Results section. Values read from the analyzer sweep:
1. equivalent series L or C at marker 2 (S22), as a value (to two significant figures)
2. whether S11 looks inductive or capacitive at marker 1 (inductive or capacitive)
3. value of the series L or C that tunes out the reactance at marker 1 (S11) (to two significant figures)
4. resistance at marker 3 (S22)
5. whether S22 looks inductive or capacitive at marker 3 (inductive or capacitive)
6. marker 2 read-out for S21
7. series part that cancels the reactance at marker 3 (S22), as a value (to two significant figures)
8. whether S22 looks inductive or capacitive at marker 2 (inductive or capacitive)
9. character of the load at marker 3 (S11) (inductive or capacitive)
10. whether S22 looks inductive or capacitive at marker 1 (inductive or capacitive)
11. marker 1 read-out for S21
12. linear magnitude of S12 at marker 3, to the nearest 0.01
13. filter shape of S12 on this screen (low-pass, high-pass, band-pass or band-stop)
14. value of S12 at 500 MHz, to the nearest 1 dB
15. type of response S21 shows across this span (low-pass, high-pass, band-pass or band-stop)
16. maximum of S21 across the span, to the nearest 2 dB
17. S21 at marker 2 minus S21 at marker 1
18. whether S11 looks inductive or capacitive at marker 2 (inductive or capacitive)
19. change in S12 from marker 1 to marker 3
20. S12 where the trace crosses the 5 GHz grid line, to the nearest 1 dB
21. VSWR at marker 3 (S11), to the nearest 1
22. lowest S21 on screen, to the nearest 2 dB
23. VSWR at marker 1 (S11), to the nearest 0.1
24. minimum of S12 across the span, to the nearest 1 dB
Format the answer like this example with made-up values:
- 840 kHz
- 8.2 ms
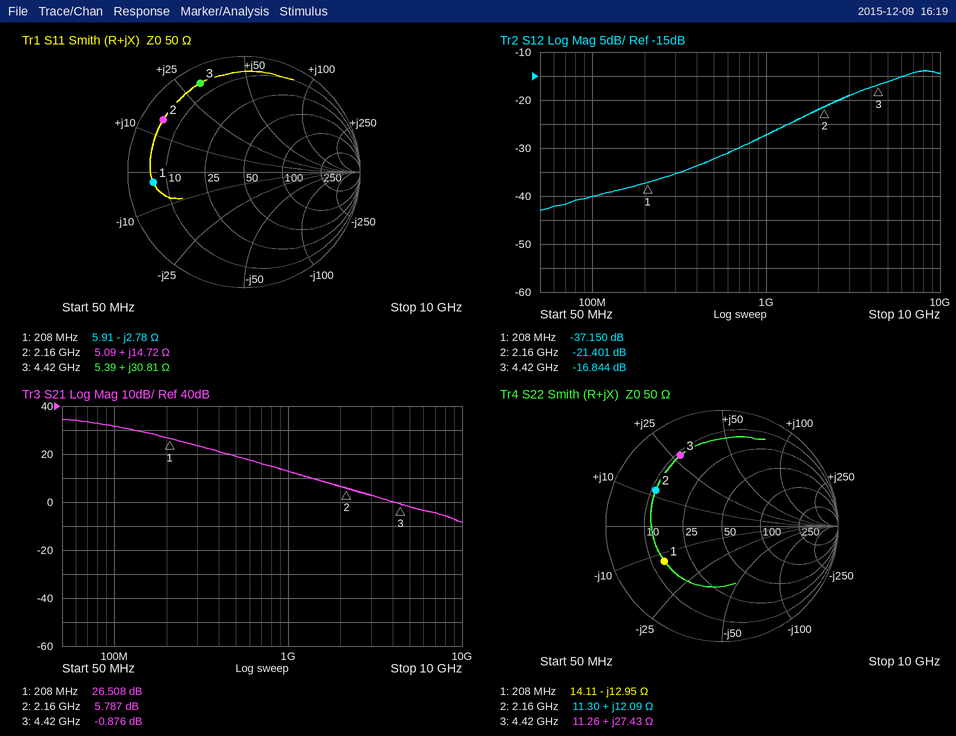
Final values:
- 890 pH
- capacitive
- 2.1 nH
- 11.26 Ω
- inductive
- 5.787 dB
- 1.3 pF
- inductive
- inductive
- capacitive
- 26.508 dB
- 0.14
- high-pass
- -32 dB
- low-pass
- 34 dB
- -20.721 dB
- inductive
- 20.306 dB
- -16 dB
- 13
- -8 dB
- 8.5
- -43 dB
